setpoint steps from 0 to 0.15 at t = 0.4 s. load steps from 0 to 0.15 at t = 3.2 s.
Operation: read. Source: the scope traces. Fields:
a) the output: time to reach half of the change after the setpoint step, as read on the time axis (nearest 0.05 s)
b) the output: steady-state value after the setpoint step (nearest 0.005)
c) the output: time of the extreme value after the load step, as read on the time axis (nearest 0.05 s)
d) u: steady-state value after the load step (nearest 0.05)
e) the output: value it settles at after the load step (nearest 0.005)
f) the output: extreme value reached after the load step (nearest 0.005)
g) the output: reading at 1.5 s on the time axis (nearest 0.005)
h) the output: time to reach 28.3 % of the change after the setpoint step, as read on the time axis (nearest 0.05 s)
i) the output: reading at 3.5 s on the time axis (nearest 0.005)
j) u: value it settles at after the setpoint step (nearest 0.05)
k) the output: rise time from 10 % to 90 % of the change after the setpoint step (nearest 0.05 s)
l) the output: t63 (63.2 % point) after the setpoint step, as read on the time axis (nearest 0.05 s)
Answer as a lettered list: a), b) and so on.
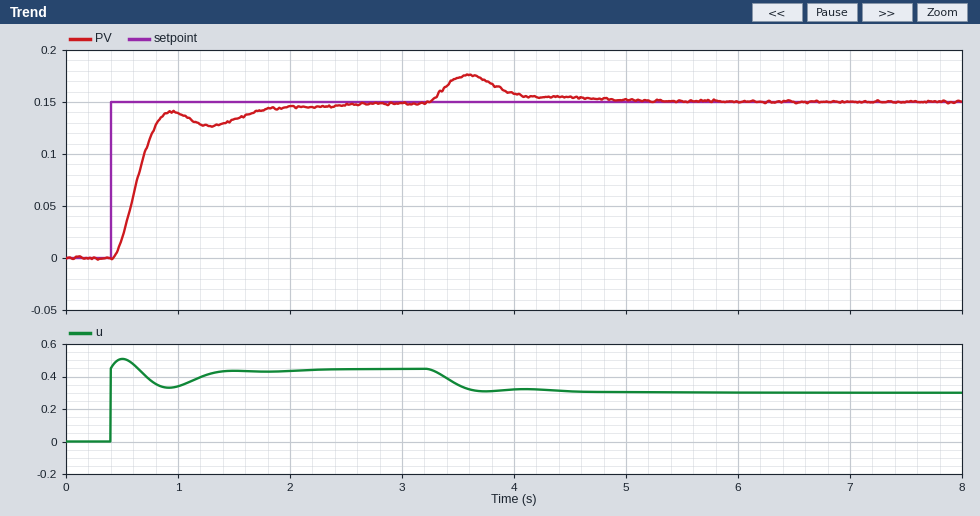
a) 0.65 s
b) 0.150
c) 3.60 s
d) 0.30
e) 0.150
f) 0.175
g) 0.135
h) 0.55 s
i) 0.175
j) 0.45
k) 0.35 s
l) 0.70 s
